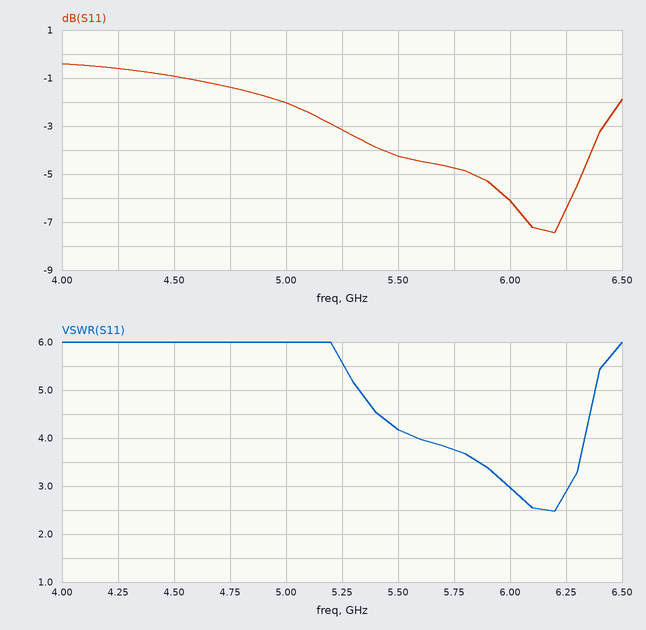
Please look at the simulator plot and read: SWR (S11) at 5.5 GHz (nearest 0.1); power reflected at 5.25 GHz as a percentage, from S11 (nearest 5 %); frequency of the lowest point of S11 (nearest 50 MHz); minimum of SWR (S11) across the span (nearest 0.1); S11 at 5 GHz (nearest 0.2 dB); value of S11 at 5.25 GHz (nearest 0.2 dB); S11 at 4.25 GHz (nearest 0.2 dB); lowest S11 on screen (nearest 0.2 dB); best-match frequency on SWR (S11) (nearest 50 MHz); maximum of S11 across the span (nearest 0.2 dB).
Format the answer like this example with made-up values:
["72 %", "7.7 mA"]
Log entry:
["4.2", "50 %", "6.20 GHz", "2.5", "-2.0 dB", "-3.2 dB", "-0.6 dB", "-7.4 dB", "6.20 GHz", "-0.4 dB"]
